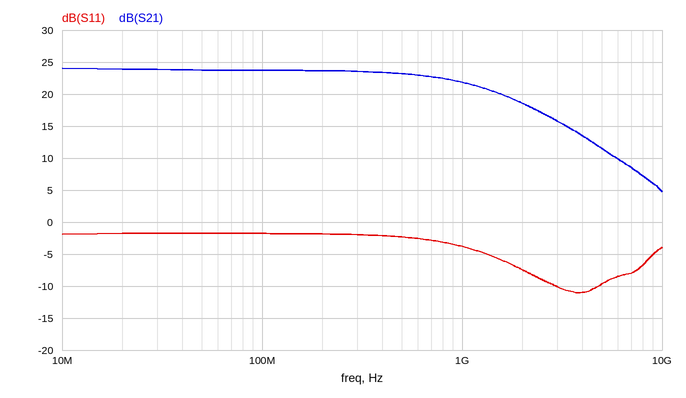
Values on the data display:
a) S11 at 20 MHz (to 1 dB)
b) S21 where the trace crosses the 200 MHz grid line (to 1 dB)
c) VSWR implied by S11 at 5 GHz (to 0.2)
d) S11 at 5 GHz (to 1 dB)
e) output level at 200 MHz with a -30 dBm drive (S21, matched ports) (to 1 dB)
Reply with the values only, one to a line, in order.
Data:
-2 dB
24 dB
2.0
-10 dB
-6 dBm
